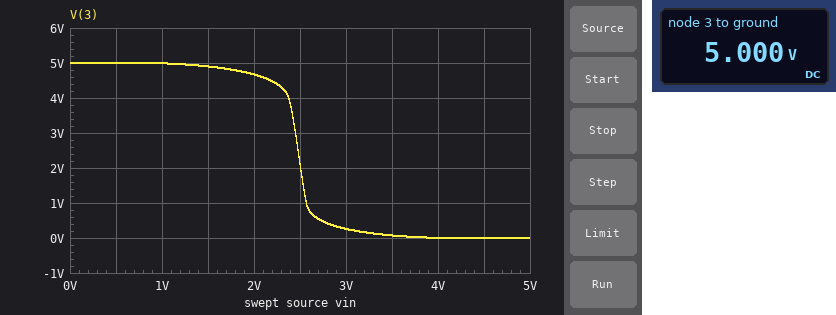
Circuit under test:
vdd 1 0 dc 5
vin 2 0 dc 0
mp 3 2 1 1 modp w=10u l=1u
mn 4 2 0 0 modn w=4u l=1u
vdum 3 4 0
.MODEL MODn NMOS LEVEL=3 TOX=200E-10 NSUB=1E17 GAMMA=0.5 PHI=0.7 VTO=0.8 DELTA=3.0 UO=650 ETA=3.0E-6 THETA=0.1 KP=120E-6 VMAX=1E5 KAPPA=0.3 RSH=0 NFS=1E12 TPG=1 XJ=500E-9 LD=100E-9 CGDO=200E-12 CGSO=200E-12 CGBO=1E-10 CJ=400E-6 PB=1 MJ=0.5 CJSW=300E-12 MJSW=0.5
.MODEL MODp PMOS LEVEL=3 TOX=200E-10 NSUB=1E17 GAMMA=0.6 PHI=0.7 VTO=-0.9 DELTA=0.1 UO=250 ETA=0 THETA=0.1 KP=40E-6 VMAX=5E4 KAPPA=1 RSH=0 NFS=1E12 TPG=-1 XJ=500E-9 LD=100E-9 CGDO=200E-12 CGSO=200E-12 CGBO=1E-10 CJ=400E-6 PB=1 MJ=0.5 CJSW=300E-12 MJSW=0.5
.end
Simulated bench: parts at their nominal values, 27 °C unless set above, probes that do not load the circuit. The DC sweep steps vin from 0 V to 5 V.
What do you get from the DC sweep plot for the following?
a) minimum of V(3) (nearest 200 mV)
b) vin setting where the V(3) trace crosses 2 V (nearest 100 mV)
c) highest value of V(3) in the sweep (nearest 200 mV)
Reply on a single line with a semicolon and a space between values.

0 V; 2.5 V; 5.0 V
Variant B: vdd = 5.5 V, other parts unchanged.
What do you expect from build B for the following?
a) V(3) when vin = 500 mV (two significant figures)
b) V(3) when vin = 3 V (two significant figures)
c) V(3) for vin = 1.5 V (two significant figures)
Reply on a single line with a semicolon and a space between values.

5.5 V; 610 mV; 5.4 V
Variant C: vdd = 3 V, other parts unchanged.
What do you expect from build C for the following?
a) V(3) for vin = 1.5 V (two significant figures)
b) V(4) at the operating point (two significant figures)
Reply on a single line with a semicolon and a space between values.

390 mV; 3.0 V
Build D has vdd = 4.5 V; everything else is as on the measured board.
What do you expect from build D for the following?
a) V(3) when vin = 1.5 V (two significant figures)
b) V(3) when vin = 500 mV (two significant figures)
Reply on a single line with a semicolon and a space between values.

4.4 V; 4.5 V
